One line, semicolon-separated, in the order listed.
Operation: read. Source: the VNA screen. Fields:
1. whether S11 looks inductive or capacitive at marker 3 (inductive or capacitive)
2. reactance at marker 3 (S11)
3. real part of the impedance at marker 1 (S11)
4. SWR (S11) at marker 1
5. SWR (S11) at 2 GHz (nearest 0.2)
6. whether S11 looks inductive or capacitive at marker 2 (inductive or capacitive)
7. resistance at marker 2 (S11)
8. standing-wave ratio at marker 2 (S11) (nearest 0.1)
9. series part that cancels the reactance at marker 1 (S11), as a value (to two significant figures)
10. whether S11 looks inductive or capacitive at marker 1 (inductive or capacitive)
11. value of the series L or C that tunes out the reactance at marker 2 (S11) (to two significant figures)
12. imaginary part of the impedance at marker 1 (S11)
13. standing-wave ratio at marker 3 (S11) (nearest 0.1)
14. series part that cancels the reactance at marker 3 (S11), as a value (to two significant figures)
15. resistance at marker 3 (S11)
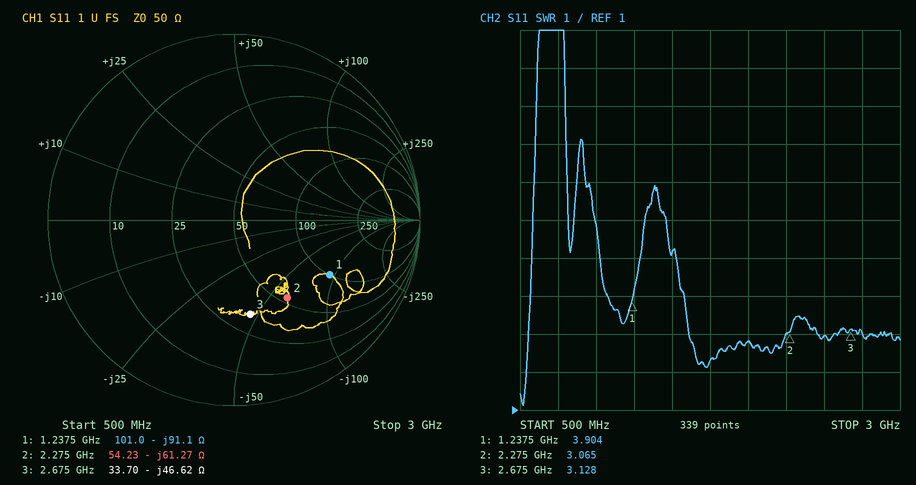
capacitive; -46.62 Ω; 101.0 Ω; 3.904; 2.8; capacitive; 54.23 Ω; 3.1; 12 nH; capacitive; 4.3 nH; -91.1 Ω; 3.1; 2.8 nH; 33.70 Ω
